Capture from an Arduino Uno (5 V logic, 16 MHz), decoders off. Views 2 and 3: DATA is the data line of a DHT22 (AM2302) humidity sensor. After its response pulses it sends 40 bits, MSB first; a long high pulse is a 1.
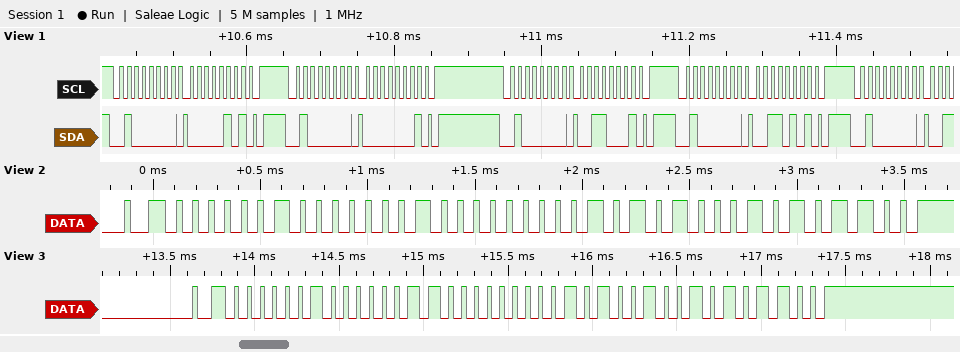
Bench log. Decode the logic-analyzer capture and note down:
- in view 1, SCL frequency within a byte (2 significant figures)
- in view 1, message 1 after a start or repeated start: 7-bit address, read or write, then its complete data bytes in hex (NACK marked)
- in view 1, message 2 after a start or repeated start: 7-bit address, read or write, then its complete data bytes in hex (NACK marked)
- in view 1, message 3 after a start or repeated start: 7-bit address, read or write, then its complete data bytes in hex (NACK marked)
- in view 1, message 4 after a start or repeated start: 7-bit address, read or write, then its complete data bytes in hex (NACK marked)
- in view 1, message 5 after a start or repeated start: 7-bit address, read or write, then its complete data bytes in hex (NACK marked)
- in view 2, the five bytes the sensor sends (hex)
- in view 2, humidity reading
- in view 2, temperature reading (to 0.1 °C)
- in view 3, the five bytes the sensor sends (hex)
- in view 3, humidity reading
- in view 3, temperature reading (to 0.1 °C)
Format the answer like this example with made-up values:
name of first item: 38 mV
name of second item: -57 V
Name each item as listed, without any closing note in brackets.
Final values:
in view 1, SCL frequency within a byte: 100 kHz
in view 1, message 1 after a start or repeated start: 7-bit address, read or write, then its complete data bytes in hex: 0x20 write: 05
in view 1, message 2 after a start or repeated start: 7-bit address, read or write, then its complete data bytes in hex: 0x20 write: 01
in view 1, message 3 after a start or repeated start: 7-bit address, read or write, then its complete data bytes in hex: 0x20 write: 31
in view 1, message 4 after a start or repeated start: 7-bit address, read or write, then its complete data bytes in hex: 0x20 write: 35
in view 1, message 5 after a start or repeated start: 7-bit address, read or write, then its complete data bytes in hex: 0x20 write
in view 2, the five bytes the sensor sends: 02 02 00 A8 AC
in view 2, humidity reading: 51.4 %
in view 2, temperature reading: 16.8 °C
in view 3, the five bytes the sensor sends: 02 06 00 A4 AC
in view 3, humidity reading: 51.8 %
in view 3, temperature reading: 16.4 °C
